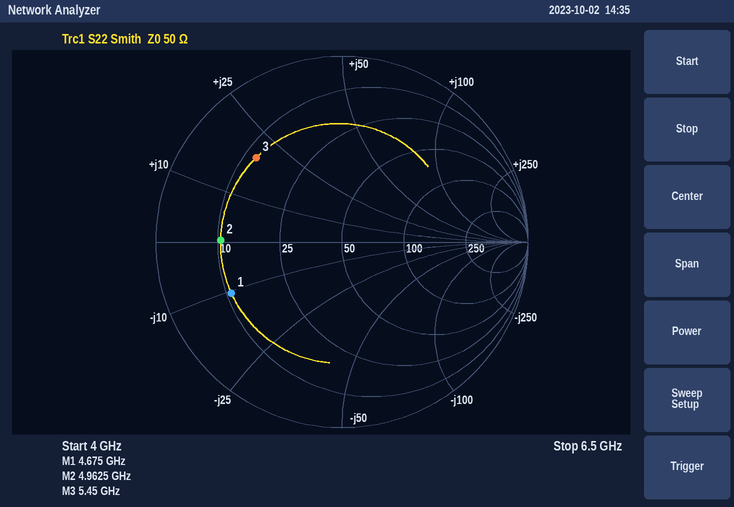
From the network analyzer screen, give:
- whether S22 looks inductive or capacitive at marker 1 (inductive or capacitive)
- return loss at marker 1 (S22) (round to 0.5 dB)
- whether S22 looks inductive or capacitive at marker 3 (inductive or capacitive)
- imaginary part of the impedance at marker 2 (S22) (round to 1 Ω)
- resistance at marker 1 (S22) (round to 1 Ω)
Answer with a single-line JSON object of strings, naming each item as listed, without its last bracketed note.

{"whether S22 looks inductive or capacitive at marker 1": "capacitive", "return loss at marker 1 (S22)": "3.5 dB", "whether S22 looks inductive or capacitive at marker 3": "inductive", "imaginary part of the impedance at marker 2 (S22)": "0 Ω", "resistance at marker 1 (S22)": "11 Ω"}
